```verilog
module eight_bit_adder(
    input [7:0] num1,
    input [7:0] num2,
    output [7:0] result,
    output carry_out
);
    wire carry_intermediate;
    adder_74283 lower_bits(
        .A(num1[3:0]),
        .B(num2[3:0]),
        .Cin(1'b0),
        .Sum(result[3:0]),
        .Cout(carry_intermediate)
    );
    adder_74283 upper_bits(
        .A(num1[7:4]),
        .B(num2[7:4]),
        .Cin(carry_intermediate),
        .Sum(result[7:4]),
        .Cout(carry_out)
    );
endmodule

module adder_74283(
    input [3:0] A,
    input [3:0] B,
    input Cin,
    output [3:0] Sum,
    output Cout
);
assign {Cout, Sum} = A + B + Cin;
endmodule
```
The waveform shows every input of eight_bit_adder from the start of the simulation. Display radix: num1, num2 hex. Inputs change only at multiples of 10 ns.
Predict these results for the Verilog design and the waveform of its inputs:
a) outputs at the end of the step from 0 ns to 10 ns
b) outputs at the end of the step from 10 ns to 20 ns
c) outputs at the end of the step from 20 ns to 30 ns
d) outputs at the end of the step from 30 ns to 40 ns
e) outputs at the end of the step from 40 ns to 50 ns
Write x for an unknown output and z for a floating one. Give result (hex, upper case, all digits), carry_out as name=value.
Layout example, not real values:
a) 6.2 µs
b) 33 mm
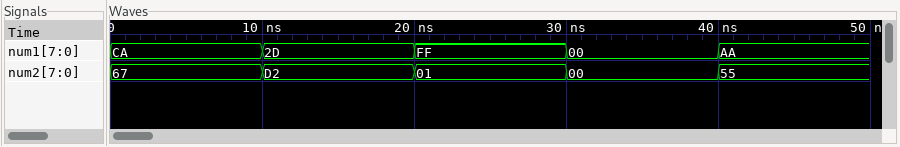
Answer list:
a) result=31, carry_out=1
b) result=FF, carry_out=0
c) result=00, carry_out=1
d) result=00, carry_out=0
e) result=FF, carry_out=0
